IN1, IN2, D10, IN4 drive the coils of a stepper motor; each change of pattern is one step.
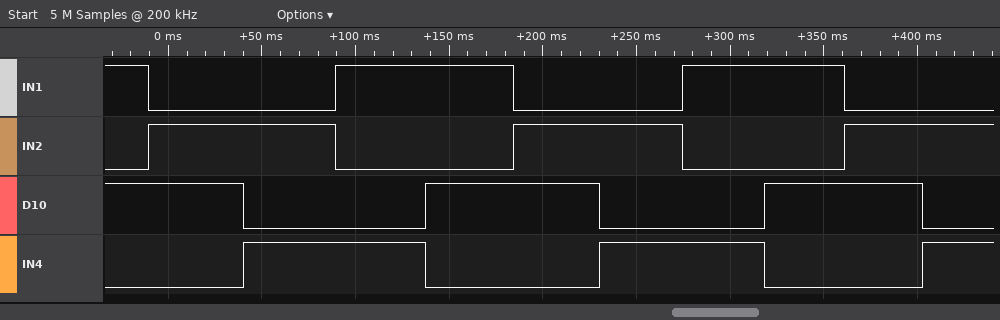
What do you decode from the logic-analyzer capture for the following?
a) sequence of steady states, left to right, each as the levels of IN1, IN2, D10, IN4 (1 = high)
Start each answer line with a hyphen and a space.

- 1010 0110 0101 1001 1010 0110 0101 1001 1010 0110 0101
